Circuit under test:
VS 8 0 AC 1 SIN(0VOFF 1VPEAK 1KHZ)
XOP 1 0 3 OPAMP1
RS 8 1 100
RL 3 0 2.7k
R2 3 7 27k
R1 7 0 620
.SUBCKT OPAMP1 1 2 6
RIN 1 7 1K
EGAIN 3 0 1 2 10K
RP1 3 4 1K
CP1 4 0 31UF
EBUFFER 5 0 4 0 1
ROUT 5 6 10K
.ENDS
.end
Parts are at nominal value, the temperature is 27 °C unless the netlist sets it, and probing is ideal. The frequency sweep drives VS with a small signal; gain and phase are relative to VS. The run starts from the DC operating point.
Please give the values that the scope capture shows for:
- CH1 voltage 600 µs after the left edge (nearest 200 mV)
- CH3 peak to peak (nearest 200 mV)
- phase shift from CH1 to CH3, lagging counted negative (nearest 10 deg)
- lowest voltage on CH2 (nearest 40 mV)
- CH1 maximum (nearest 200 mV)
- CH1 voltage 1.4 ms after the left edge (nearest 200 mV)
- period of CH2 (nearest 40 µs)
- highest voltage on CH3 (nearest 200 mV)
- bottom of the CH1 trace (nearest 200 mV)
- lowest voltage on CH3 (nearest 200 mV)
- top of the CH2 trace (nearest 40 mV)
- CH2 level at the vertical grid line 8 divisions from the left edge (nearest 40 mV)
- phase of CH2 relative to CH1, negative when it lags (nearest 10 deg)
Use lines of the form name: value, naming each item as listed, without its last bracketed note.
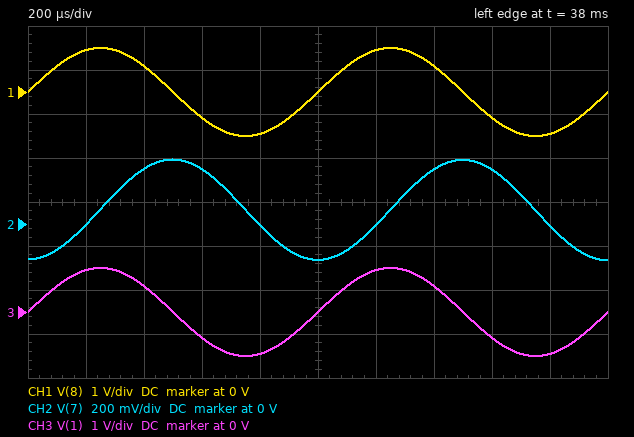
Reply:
CH1 voltage 600 µs after the left edge: -600 mV
CH3 peak to peak: 2.0 V
phase shift from CH1 to CH3, lagging counted negative: 0 deg
lowest voltage on CH2: -160 mV
CH1 maximum: 1.0 V
CH1 voltage 1.4 ms after the left edge: 600 mV
period of CH2: 1.00 ms
highest voltage on CH3: 1.0 V
bottom of the CH1 trace: -1.0 V
lowest voltage on CH3: -1.0 V
top of the CH2 trace: 280 mV
CH2 level at the vertical grid line 8 divisions from the left edge: 240 mV
phase of CH2 relative to CH1, negative when it lags: -90 deg
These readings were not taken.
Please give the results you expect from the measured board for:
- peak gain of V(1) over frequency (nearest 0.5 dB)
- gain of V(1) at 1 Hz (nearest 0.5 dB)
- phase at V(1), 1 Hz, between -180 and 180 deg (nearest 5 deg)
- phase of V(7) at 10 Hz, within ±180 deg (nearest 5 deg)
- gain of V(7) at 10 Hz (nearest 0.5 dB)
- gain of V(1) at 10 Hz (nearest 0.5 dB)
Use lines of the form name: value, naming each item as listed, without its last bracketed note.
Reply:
peak gain of V(1) over frequency: 0 dB
gain of V(1) at 1 Hz: 0 dB
phase at V(1), 1 Hz, between -180 and 180 deg: 0 deg
phase of V(7) at 10 Hz, within ±180 deg: -65 deg
gain of V(7) at 10 Hz: 26.0 dB
gain of V(1) at 10 Hz: 0 dB
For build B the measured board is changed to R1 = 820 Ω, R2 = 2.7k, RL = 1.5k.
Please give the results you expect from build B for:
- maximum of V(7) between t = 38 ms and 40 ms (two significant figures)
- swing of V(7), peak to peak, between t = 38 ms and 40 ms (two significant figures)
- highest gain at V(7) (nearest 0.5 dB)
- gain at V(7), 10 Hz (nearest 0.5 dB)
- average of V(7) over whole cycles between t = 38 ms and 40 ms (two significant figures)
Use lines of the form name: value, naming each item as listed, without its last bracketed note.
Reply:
maximum of V(7) between t = 38 ms and 40 ms: 1.5 V
swing of V(7), peak to peak, between t = 38 ms and 40 ms: 2.3 V
highest gain at V(7): 47.0 dB
gain at V(7), 10 Hz: 40.0 dB
average of V(7) over whole cycles between t = 38 ms and 40 ms: 330 mV
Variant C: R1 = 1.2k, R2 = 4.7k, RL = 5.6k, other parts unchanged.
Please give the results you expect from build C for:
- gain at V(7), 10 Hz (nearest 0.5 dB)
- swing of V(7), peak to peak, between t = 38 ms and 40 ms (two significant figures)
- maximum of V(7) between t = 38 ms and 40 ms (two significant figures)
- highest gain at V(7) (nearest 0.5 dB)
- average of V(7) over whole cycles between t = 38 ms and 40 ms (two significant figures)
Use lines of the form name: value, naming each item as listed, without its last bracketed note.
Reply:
gain at V(7), 10 Hz: 46.5 dB
swing of V(7), peak to peak, between t = 38 ms and 40 ms: 4.7 V
maximum of V(7) between t = 38 ms and 40 ms: 3.0 V
highest gain at V(7): 53.0 dB
average of V(7) over whole cycles between t = 38 ms and 40 ms: 670 mV
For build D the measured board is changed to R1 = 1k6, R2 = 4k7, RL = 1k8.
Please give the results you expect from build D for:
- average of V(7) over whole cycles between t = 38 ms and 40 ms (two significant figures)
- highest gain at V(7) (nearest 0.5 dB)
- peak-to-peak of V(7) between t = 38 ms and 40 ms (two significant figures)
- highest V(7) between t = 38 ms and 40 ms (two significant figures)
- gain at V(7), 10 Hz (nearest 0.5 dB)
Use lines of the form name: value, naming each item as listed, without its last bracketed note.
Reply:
average of V(7) over whole cycles between t = 38 ms and 40 ms: 460 mV
highest gain at V(7): 50.0 dB
peak-to-peak of V(7) between t = 38 ms and 40 ms: 3.2 V
highest V(7) between t = 38 ms and 40 ms: 2.1 V
gain at V(7), 10 Hz: 43.0 dB
